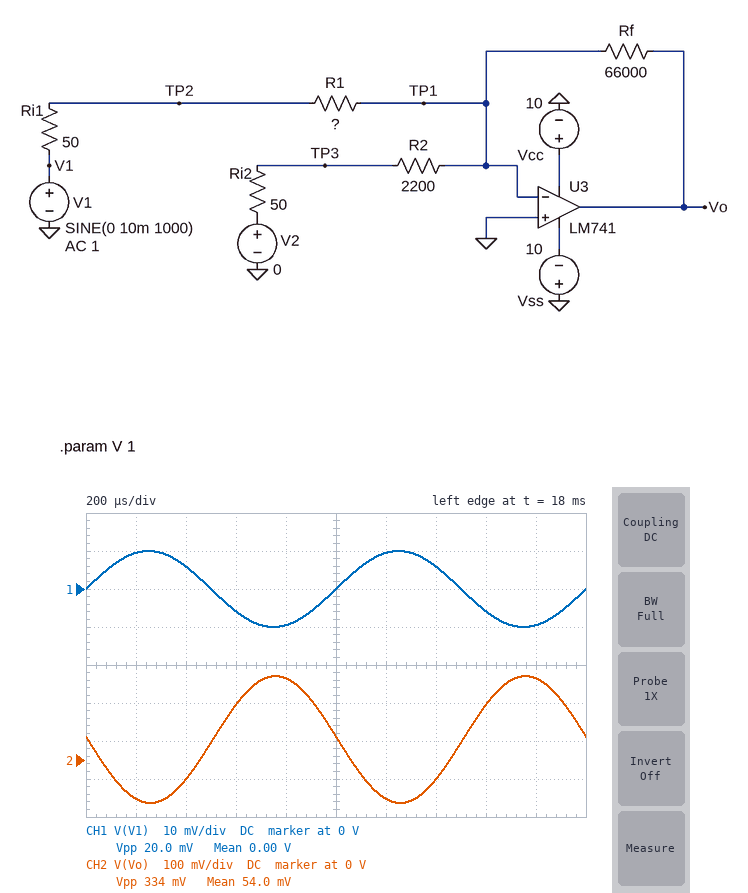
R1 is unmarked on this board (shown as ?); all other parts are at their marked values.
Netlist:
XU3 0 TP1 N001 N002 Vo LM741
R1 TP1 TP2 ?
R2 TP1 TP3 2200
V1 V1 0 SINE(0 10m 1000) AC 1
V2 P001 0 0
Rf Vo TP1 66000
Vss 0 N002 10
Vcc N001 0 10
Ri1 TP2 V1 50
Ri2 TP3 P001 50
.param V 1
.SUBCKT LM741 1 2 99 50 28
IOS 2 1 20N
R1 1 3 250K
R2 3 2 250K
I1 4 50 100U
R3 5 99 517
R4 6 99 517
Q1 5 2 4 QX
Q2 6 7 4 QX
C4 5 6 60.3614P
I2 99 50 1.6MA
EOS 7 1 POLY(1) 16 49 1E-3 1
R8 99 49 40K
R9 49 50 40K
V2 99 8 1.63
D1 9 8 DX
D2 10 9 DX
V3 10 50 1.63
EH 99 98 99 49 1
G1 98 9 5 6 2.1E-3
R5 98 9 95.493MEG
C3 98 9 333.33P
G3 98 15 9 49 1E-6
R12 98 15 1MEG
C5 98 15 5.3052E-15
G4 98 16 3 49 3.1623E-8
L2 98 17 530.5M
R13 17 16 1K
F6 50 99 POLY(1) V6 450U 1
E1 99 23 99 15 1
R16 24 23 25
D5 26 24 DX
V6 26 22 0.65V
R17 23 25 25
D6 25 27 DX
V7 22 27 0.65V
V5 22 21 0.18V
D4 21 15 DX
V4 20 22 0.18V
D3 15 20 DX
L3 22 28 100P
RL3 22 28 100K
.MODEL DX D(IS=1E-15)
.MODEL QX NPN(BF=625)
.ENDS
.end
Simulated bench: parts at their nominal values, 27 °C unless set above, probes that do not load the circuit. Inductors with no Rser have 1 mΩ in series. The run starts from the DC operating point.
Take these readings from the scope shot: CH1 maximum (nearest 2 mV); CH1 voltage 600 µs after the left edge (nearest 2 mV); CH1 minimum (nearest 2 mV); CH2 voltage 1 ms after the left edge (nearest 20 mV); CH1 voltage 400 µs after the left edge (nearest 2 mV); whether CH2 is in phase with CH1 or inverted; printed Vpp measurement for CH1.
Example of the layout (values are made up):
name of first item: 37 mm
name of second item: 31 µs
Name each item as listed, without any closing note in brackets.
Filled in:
CH1 maximum: 10 mV
CH1 voltage 600 µs after the left edge: -6 mV
CH1 minimum: -10 mV
CH2 voltage 1 ms after the left edge: 60 mV
CH1 voltage 400 µs after the left edge: 6 mV
whether CH2 is in phase with CH1 or inverted: inverted
printed Vpp measurement for CH1: 20.0 mV
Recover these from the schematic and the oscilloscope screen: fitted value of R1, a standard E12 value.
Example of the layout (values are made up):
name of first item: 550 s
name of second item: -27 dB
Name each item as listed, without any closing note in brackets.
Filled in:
fitted value of R1, a standard E12 value: 3.9 kΩ
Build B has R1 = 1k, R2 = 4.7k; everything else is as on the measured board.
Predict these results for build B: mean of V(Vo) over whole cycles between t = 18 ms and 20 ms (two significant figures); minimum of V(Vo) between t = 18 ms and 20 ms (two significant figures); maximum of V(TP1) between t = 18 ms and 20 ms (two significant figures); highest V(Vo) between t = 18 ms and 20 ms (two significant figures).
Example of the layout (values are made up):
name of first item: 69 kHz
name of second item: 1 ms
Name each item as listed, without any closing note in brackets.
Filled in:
mean of V(Vo) over whole cycles between t = 18 ms and 20 ms: 84 mV
minimum of V(Vo) between t = 18 ms and 20 ms: -540 mV
maximum of V(TP1) between t = 18 ms and 20 ms: 1.6 mV
highest V(Vo) between t = 18 ms and 20 ms: 710 mV
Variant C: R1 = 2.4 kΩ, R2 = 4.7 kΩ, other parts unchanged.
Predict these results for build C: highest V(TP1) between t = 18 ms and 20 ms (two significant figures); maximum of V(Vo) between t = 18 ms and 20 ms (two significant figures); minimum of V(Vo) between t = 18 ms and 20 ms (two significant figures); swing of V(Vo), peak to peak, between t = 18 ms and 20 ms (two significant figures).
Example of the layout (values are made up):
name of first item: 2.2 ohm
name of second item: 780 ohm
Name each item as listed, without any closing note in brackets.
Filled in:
highest V(TP1) between t = 18 ms and 20 ms: 1.3 mV
maximum of V(Vo) between t = 18 ms and 20 ms: 320 mV
minimum of V(Vo) between t = 18 ms and 20 ms: -220 mV
swing of V(Vo), peak to peak, between t = 18 ms and 20 ms: 540 mV
